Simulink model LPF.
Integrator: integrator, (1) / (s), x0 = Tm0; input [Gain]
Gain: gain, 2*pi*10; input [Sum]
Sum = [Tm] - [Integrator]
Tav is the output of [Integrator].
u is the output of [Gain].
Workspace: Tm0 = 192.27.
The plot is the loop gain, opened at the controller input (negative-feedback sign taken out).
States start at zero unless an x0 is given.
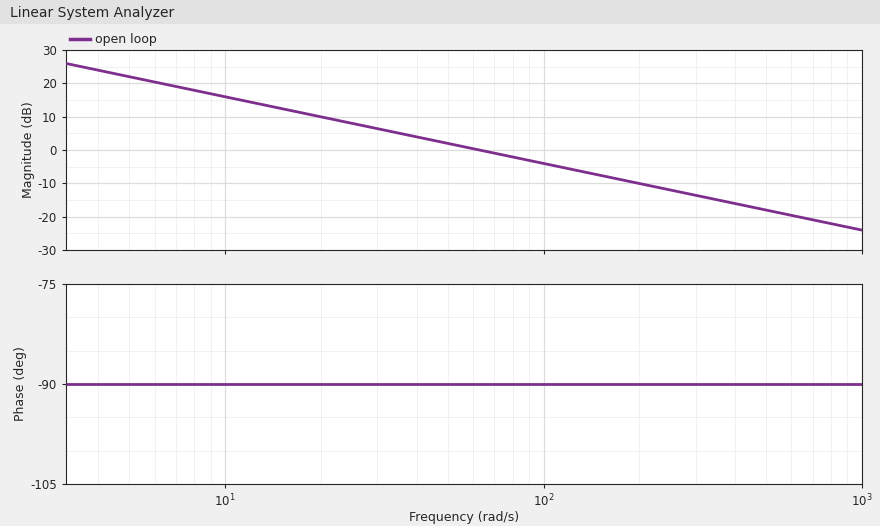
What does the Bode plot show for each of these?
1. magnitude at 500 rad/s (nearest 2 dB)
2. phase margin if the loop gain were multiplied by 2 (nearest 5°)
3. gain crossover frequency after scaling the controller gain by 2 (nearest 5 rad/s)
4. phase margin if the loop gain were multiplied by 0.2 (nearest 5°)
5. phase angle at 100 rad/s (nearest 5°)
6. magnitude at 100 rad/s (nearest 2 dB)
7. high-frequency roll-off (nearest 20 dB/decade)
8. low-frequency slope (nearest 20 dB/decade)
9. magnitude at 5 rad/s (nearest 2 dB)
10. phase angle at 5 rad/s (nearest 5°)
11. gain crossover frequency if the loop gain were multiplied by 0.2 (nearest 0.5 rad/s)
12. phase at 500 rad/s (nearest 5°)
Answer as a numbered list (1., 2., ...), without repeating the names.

1. -18 dB
2. 90°
3. 125 rad/s
4. 90°
5. -90°
6. -4 dB
7. -20 dB/decade
8. -20 dB/decade
9. 22 dB
10. -90°
11. 12.5 rad/s
12. -90°
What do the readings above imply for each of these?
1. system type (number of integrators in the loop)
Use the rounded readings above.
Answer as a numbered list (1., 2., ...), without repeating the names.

1. 1
